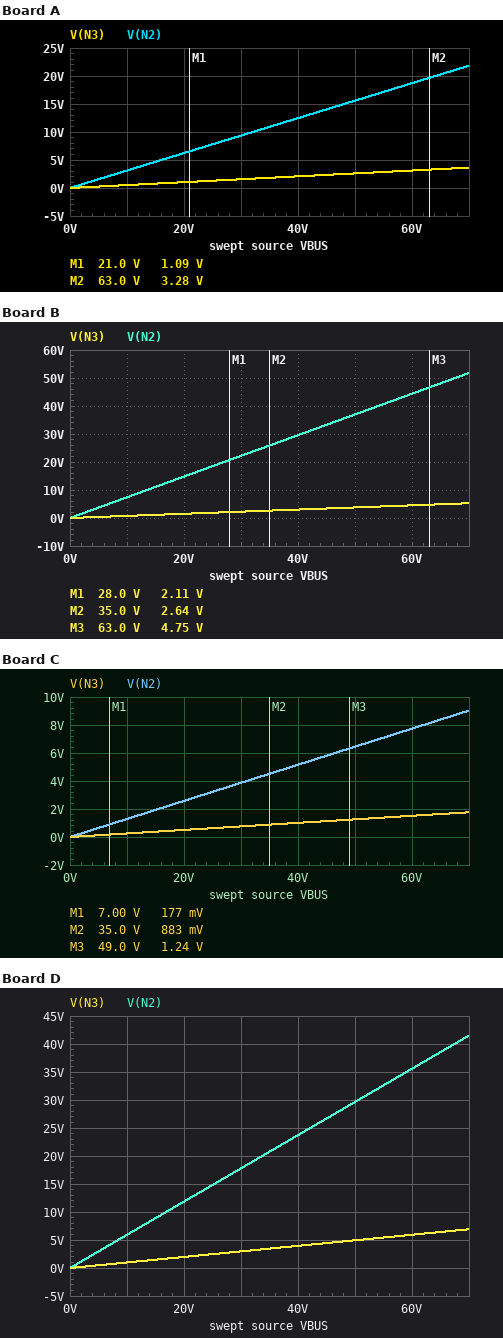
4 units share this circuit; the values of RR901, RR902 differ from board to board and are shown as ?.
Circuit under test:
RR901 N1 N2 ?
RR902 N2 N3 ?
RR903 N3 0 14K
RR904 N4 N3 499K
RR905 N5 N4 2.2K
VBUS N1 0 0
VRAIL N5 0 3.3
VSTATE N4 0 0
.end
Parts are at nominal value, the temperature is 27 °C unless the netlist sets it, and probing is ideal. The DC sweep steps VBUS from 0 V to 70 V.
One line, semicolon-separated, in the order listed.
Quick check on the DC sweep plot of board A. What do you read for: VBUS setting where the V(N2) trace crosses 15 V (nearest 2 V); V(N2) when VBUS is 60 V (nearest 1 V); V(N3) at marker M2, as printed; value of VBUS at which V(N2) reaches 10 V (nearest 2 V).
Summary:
48 V; 19 V; 3.28 V; 32 V
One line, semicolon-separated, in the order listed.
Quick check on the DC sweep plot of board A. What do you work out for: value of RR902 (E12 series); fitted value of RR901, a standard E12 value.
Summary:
68 kΩ; 180 kΩ
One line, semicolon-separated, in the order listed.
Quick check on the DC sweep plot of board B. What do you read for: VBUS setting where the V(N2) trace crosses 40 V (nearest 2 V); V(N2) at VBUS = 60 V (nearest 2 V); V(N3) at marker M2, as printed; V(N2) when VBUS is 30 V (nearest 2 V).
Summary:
54 V; 44 V; 2.64 V; 22 V
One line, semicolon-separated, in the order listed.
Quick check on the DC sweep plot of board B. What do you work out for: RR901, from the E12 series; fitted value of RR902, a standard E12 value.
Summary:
47 kΩ; 120 kΩ
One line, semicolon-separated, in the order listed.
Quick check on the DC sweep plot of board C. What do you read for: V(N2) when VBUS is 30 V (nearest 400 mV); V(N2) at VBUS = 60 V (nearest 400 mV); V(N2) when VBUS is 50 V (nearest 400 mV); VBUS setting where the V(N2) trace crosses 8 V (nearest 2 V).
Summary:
4.0 V; 7.6 V; 6.4 V; 62 V
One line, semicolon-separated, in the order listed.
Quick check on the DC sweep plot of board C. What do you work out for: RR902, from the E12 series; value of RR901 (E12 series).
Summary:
56 kΩ; 470 kΩ
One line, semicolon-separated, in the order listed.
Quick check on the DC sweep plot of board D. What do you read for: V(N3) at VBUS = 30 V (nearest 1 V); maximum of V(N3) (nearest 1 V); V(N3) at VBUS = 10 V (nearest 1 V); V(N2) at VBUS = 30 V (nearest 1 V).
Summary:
3 V; 7 V; 1 V; 18 V
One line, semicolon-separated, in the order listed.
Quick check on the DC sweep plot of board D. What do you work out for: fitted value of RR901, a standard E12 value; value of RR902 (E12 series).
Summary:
56 kΩ; 68 kΩ
